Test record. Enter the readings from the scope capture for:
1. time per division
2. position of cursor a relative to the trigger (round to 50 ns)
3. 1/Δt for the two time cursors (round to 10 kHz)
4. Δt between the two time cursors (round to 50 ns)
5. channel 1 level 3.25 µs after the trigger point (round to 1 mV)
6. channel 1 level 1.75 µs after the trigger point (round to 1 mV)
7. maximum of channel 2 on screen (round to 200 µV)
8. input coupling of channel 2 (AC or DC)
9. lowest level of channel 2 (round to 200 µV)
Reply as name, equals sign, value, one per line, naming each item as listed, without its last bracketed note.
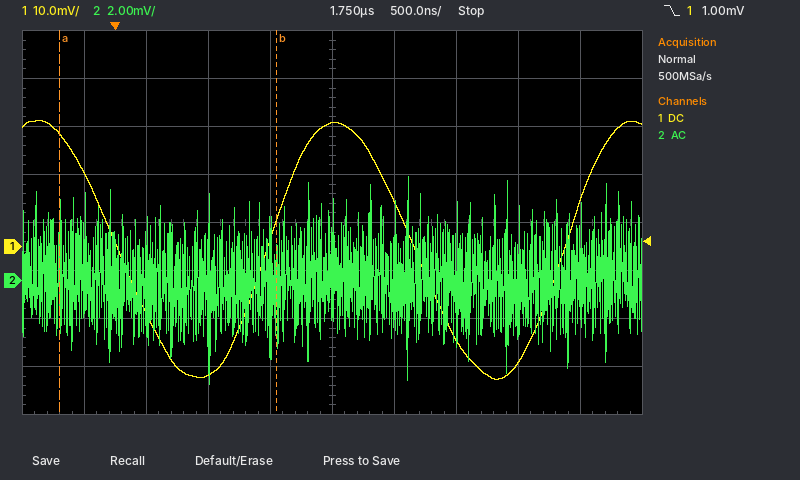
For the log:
time per division = 500 ns
position of cursor a relative to the trigger = -450 ns
1/Δt for the two time cursors = 570 kHz
Δt between the two time cursors = 1.75 µs
channel 1 level 3.25 µs after the trigger point = -24 mV
channel 1 level 1.75 µs after the trigger point = 26 mV
maximum of channel 2 on screen = 4.4 mV
input coupling of channel 2 = AC
lowest level of channel 2 = -4.4 mV
